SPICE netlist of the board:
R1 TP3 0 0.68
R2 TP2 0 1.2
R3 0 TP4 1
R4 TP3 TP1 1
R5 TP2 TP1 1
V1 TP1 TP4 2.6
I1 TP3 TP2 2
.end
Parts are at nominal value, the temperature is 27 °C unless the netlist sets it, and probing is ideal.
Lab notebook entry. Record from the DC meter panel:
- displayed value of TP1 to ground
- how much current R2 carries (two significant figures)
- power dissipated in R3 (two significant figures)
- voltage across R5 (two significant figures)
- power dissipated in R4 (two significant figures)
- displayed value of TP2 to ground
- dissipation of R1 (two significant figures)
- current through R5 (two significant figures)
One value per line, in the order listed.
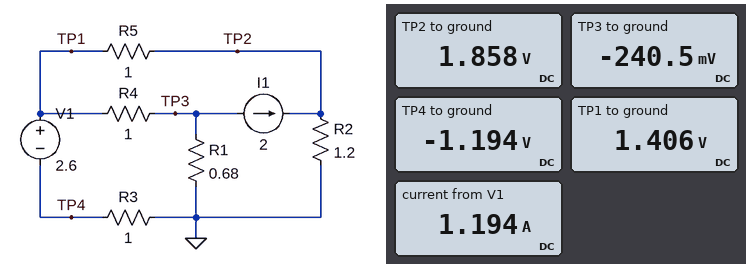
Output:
1.406 V
1.5 A
1.4 W
450 mV
2.7 W
1.858 V
85 mW
450 mA
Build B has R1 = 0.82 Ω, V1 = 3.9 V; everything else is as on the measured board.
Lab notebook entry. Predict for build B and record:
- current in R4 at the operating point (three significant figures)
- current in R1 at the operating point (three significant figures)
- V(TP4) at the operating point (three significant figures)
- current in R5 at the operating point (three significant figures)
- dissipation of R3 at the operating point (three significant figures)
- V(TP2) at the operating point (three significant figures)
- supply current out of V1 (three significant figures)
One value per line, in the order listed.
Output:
2.02 A
22.4 mA
-1.86 V
163 mA
3.46 W
2.20 V
1.86 A
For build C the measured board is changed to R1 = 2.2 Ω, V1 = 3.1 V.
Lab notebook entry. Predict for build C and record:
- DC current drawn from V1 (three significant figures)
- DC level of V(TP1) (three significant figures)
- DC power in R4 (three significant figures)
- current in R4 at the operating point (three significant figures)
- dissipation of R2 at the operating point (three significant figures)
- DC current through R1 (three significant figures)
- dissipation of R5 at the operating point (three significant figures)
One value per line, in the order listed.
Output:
1.51 A
1.59 V
3.51 W
1.87 A
3.20 W
127 mA
134 mW
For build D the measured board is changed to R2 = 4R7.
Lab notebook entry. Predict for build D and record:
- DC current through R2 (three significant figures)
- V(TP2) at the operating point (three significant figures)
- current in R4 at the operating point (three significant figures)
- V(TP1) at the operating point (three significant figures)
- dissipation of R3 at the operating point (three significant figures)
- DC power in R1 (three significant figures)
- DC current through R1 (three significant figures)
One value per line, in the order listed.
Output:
692 mA
3.25 V
1.97 A
1.94 V
432 mW
796 µW
34.2 mA
